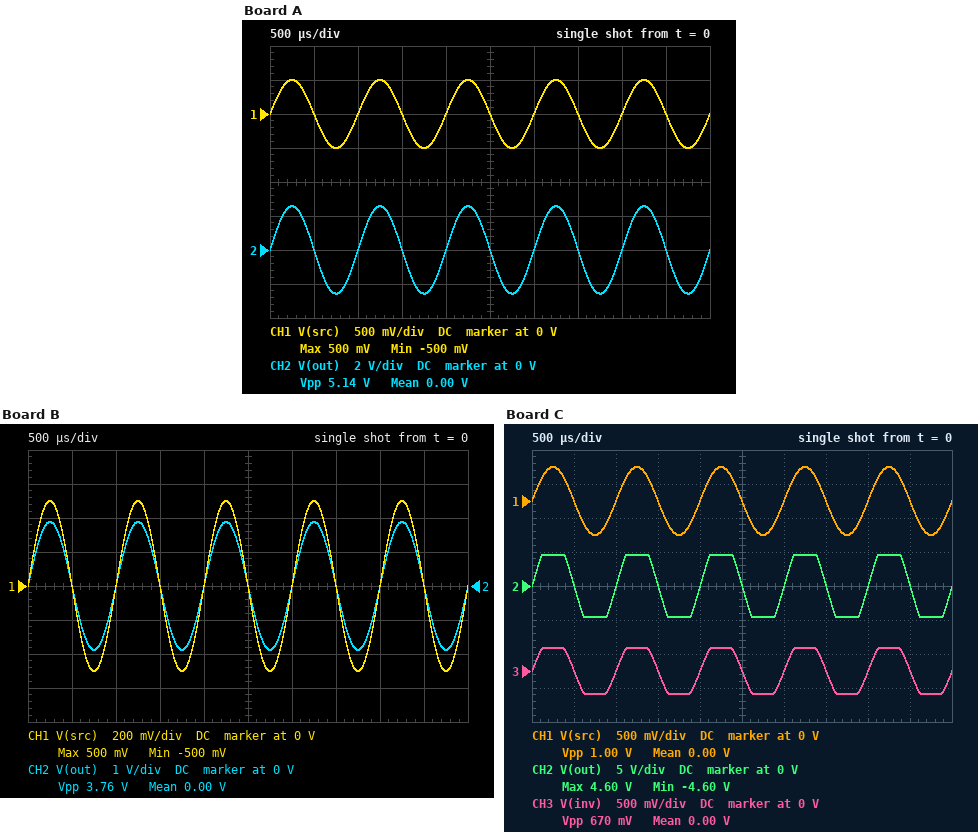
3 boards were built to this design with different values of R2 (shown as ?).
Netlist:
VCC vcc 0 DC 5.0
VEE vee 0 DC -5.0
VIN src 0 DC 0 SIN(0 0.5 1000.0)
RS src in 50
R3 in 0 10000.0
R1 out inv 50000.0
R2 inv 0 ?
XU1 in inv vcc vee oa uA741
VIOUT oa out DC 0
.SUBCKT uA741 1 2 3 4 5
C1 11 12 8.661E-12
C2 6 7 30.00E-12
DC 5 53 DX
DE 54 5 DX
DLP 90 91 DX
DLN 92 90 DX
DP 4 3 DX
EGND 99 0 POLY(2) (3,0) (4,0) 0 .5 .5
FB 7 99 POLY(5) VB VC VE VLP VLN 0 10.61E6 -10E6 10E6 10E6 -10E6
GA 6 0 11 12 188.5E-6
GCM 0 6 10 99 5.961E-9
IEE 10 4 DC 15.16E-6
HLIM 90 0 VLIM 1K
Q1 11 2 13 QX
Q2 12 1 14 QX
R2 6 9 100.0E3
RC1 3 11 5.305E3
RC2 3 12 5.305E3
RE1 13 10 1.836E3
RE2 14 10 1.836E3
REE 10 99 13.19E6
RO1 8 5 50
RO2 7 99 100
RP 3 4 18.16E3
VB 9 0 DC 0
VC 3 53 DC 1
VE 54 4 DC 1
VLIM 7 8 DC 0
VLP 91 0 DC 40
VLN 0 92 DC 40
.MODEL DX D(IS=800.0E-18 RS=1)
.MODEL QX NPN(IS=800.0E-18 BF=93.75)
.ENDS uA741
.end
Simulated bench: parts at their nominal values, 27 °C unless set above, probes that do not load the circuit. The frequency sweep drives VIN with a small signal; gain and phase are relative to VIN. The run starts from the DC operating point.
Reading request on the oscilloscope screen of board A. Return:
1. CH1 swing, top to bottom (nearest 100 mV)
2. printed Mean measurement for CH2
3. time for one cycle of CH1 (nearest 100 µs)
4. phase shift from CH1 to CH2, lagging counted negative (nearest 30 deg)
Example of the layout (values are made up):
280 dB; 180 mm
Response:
1.0 V; 0.00 V; 1.0 ms; 0 deg
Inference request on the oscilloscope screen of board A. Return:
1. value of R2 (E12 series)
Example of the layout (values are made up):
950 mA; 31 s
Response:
12 kΩ
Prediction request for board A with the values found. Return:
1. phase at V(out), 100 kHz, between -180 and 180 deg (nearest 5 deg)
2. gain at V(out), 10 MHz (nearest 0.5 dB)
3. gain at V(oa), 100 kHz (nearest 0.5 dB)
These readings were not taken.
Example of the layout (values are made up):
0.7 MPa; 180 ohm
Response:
-30 deg; -35.5 dB; 13.5 dB
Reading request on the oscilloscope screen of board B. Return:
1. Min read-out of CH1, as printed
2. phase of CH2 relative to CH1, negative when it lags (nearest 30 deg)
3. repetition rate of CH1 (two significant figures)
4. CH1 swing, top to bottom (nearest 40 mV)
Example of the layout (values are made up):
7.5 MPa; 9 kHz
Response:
-500 mV; 0 deg; 1.0 kHz; 1.00 V
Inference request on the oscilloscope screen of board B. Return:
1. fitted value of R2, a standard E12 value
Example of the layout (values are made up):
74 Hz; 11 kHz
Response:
18 kΩ
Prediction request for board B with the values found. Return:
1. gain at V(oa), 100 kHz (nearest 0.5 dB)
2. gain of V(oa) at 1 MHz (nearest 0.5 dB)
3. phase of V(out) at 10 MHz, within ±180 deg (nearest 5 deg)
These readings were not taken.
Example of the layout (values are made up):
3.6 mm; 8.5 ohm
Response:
11.0 dB; -0.5 dB; -170 deg
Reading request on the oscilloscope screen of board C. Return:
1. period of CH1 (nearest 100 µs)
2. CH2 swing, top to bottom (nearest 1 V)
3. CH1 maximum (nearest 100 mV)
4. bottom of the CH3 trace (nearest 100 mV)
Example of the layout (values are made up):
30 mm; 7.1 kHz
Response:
1.0 ms; 9 V; 500 mV; -300 mV
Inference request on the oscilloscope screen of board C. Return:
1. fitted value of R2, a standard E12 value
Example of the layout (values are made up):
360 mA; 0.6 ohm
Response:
3.9 kΩ
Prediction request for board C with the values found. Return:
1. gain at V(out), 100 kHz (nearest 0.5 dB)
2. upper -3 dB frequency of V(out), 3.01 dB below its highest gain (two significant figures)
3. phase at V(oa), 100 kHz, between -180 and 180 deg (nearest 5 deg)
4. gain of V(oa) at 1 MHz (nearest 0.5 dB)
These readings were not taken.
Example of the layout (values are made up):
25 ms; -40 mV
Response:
18.5 dB; 75 kHz; -55 deg; -1.0 dB
